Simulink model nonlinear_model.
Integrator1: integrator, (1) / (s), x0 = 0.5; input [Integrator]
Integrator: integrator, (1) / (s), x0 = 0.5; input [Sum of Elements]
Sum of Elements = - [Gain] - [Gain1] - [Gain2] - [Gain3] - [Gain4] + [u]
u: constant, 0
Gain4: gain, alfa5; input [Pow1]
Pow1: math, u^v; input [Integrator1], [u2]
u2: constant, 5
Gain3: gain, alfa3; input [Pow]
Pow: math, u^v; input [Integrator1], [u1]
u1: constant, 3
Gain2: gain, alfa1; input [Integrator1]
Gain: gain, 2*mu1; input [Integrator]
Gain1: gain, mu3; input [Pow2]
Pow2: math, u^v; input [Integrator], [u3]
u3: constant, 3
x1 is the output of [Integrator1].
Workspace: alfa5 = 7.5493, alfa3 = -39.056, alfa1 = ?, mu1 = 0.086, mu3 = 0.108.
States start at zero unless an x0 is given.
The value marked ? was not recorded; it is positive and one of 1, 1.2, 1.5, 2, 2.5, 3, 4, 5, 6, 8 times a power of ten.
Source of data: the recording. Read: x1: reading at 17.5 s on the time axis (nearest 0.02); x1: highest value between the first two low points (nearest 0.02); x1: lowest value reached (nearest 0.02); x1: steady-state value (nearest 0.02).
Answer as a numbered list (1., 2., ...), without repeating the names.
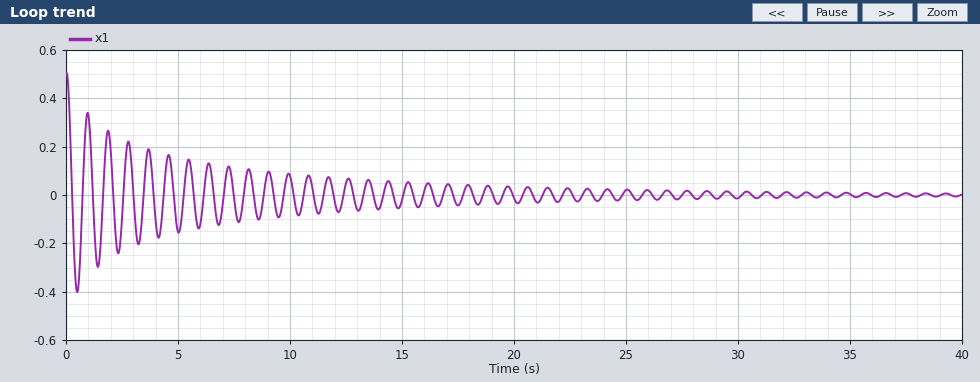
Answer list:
1. -0.04
2. 0.34
3. -0.40
4. 0.00
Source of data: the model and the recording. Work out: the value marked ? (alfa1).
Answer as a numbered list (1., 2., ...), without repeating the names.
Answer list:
1. 50
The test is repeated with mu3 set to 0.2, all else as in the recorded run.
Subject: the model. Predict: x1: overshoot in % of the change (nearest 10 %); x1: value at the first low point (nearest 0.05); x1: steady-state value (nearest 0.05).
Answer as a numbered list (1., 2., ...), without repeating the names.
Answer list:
1. 70 %
2. -0.35
3. 0.00
